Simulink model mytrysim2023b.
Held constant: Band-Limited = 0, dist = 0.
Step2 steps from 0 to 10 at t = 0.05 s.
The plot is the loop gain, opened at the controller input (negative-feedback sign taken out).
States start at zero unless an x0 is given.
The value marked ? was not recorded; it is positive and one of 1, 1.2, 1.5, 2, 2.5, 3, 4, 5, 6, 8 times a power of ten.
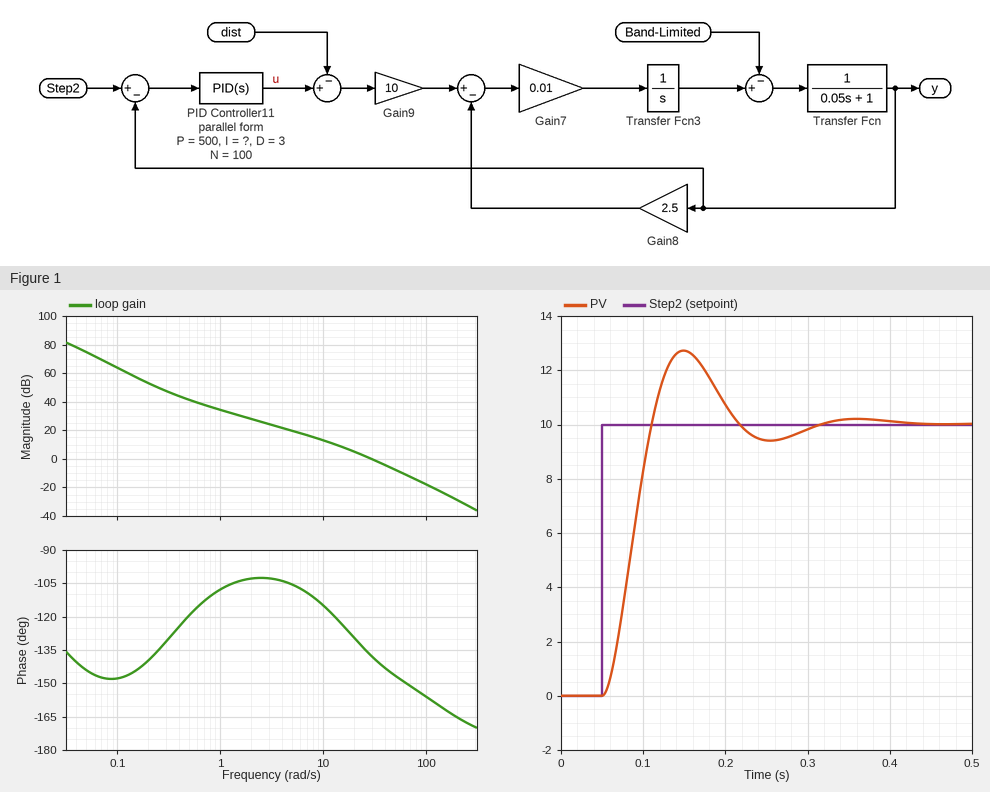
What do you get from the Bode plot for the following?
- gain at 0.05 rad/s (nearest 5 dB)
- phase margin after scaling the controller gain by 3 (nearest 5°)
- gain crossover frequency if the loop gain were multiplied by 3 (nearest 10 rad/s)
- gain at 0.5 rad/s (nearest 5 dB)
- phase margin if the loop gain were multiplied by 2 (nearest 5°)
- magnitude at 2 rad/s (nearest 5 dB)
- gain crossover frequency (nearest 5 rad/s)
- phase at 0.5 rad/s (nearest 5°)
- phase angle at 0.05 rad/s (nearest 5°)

75 dB
30°
60 rad/s
40 dB
35°
30 dB
30 rad/s
-120°
-145°
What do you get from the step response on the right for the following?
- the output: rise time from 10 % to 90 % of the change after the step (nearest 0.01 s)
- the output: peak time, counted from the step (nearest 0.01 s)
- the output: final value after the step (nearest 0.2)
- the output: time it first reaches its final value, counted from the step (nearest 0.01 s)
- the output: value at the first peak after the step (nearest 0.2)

0.04 s
0.10 s
10.0
0.06 s
12.8
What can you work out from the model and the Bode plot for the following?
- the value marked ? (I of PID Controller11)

150
